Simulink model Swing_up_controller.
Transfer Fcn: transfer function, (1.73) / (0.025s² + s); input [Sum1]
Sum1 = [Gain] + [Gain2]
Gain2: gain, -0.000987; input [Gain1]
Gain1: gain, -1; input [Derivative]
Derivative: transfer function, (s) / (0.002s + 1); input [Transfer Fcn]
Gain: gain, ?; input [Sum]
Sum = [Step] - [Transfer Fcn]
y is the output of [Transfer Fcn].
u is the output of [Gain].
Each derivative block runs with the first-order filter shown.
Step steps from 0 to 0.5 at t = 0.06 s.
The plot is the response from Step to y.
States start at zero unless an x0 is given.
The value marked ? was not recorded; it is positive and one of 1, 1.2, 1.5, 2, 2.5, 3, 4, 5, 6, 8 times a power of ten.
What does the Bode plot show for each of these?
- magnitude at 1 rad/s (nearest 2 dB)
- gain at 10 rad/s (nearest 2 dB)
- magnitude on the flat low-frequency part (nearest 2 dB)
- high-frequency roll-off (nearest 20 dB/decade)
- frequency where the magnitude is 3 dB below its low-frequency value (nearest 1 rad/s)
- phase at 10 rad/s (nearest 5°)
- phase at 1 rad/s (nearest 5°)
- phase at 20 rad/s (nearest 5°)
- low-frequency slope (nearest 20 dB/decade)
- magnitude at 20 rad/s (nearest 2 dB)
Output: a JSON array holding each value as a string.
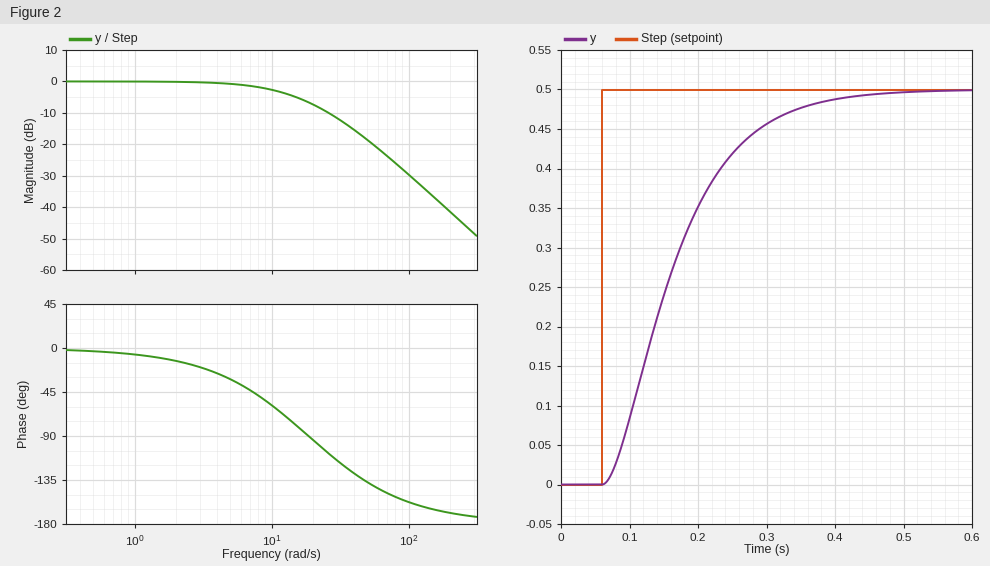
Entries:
["0 dB", "-2 dB", "0 dB", "-40 dB/decade", "11 rad/s", "-60°", "-5°", "-95°", "0 dB/decade", "-8 dB"]
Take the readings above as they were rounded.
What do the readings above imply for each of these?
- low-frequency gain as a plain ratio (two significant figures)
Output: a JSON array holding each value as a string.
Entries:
["1.0"]
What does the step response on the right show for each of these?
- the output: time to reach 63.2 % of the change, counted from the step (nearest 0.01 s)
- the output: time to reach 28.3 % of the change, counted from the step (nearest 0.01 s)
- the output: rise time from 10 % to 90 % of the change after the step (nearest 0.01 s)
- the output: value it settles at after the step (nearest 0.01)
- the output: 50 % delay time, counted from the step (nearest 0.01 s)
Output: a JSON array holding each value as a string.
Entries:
["0.12 s", "0.06 s", "0.20 s", "0.50", "0.09 s"]
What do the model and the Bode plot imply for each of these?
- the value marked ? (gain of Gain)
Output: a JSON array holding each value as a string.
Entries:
["5"]
